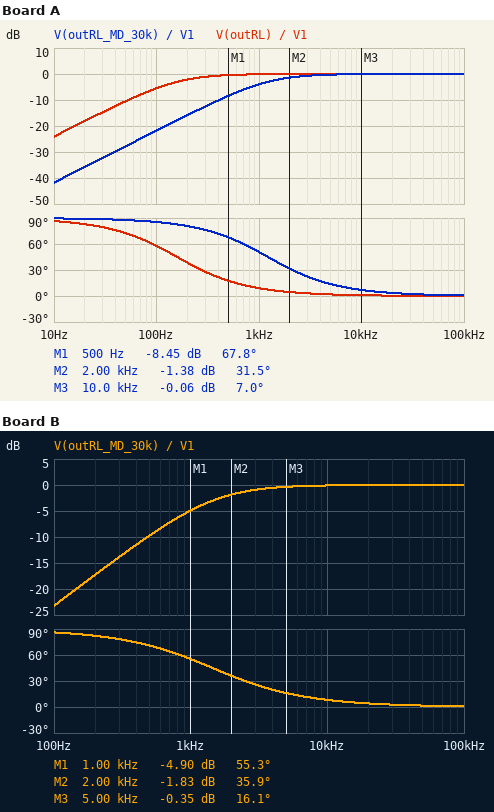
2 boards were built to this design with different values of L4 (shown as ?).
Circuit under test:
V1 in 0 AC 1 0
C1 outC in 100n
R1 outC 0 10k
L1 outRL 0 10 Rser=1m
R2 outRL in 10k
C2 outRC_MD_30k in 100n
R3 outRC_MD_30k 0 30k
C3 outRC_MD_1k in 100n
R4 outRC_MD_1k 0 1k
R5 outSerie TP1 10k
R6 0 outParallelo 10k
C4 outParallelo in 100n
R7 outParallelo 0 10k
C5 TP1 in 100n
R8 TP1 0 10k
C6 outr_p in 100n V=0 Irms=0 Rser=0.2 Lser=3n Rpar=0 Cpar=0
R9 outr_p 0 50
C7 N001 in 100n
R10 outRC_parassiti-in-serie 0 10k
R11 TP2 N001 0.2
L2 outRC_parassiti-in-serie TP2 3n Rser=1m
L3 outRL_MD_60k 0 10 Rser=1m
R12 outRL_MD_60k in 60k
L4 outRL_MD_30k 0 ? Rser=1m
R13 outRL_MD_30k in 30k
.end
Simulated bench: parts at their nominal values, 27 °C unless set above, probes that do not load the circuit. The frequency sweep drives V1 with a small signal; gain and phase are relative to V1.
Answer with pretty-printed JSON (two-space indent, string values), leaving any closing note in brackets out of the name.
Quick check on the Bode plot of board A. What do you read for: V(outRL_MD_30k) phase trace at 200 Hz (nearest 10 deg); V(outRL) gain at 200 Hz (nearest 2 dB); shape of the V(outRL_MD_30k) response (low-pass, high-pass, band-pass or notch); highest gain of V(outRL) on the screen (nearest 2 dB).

{
  "V(outRL_MD_30k) phase trace at 200 Hz": "80 deg",
  "V(outRL) gain at 200 Hz": "-2 dB",
  "shape of the V(outRL_MD_30k) response": "high-pass",
  "highest gain of V(outRL) on the screen": "0 dB"
}
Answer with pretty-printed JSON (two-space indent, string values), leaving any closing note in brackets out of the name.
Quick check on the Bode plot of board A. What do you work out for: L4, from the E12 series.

{
  "L4, from the E12 series": "3.9 H"
}
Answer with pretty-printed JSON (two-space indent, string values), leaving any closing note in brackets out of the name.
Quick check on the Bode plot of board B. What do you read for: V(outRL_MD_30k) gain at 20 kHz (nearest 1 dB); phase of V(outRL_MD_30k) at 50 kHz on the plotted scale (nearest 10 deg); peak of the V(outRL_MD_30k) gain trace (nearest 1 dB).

{
  "V(outRL_MD_30k) gain at 20 kHz": "0 dB",
  "phase of V(outRL_MD_30k) at 50 kHz on the plotted scale": "0 deg",
  "peak of the V(outRL_MD_30k) gain trace": "0 dB"
}
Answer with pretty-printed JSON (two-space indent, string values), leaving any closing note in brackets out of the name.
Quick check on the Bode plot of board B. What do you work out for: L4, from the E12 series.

{
  "L4, from the E12 series": "3.3 H"
}
